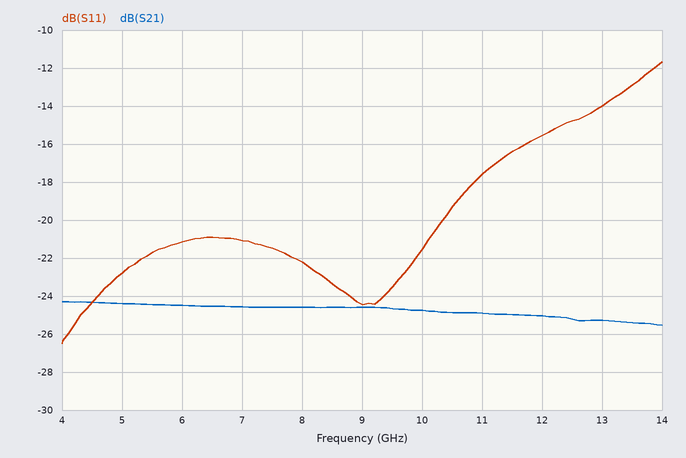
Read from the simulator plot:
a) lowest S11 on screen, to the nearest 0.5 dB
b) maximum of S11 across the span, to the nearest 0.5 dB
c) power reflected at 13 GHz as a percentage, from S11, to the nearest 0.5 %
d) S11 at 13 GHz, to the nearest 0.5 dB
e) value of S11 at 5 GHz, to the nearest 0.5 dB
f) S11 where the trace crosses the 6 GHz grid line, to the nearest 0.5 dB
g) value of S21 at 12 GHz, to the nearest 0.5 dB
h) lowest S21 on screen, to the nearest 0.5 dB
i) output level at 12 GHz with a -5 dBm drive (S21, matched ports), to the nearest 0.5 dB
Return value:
-26.5 dB
-11.5 dB
4.0 %
-14.0 dB
-23.0 dB
-21.0 dB
-25.0 dB
-25.5 dB
-30.0 dBm
